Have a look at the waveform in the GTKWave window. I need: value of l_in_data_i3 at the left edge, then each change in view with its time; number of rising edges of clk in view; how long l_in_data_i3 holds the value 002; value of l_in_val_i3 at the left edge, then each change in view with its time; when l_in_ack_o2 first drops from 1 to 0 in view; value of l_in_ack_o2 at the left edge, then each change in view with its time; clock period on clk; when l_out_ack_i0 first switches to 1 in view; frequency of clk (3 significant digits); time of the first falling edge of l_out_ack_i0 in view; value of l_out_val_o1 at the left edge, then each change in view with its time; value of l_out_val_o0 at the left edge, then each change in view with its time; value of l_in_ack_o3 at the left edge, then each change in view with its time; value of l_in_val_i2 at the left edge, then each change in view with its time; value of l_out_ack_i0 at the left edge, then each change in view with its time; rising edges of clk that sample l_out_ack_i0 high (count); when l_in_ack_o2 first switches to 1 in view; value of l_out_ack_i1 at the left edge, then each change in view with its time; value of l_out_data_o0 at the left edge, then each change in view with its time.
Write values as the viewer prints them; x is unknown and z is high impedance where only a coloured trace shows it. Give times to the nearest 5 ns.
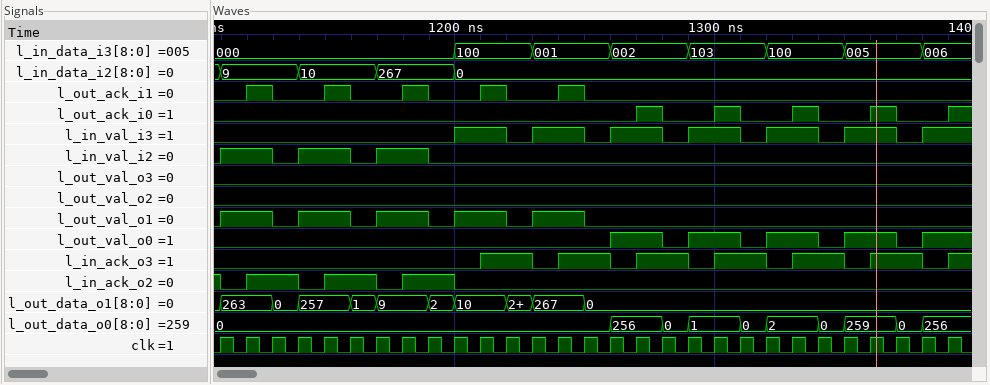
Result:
000, 100 at 1200 ns, 001 at 1230 ns, 002 at 1260 ns, 103 at 1290 ns, 100 at 1320 ns, 005 at 1350 ns, 006 at 1380 ns
29
30 ns
0, 1 at 1200 ns, 0 at 1220 ns, 1 at 1230 ns, 0 at 1250 ns, 1 at 1260 ns, 0 at 1280 ns, 1 at 1290 ns, 0 at 1310 ns, 1 at 1320 ns, 0 at 1340 ns, 1 at 1350 ns, 0 at 1370 ns, 1 at 1380 ns
1110 ns
1, 0 at 1110 ns, 1 at 1120 ns, 0 at 1140 ns, 1 at 1150 ns, 0 at 1170 ns, 1 at 1180 ns, 0 at 1200 ns
10 ns
1270 ns
100 MHz
1280 ns
0, 1 at 1110 ns, 0 at 1130 ns, 1 at 1140 ns, 0 at 1160 ns, 1 at 1170 ns, 0 at 1190 ns, 1 at 1200 ns, 0 at 1220 ns, 1 at 1230 ns, 0 at 1250 ns
0, 1 at 1260 ns, 0 at 1280 ns, 1 at 1290 ns, 0 at 1310 ns, 1 at 1320 ns, 0 at 1340 ns, 1 at 1350 ns, 0 at 1370 ns, 1 at 1380 ns
0, 1 at 1210 ns, 0 at 1230 ns, 1 at 1240 ns, 0 at 1260 ns, 1 at 1270 ns, 0 at 1290 ns, 1 at 1300 ns, 0 at 1320 ns, 1 at 1330 ns, 0 at 1350 ns, 1 at 1360 ns, 0 at 1380 ns, 1 at 1390 ns
0, 1 at 1110 ns, 0 at 1130 ns, 1 at 1140 ns, 0 at 1160 ns, 1 at 1170 ns, 0 at 1190 ns
0, 1 at 1270 ns, 0 at 1280 ns, 1 at 1300 ns, 0 at 1310 ns, 1 at 1330 ns, 0 at 1340 ns, 1 at 1360 ns, 0 at 1370 ns, 1 at 1390 ns
4
1120 ns
0, 1 at 1120 ns, 0 at 1130 ns, 1 at 1150 ns, 0 at 1160 ns, 1 at 1180 ns, 0 at 1190 ns, 1 at 1210 ns, 0 at 1220 ns, 1 at 1240 ns, 0 at 1250 ns
0, 256 at 1260 ns, 0 at 1280 ns, 1 at 1290 ns, 0 at 1310 ns, 2 at 1320 ns, 0 at 1340 ns, 259 at 1350 ns, 0 at 1370 ns, 256 at 1380 ns
